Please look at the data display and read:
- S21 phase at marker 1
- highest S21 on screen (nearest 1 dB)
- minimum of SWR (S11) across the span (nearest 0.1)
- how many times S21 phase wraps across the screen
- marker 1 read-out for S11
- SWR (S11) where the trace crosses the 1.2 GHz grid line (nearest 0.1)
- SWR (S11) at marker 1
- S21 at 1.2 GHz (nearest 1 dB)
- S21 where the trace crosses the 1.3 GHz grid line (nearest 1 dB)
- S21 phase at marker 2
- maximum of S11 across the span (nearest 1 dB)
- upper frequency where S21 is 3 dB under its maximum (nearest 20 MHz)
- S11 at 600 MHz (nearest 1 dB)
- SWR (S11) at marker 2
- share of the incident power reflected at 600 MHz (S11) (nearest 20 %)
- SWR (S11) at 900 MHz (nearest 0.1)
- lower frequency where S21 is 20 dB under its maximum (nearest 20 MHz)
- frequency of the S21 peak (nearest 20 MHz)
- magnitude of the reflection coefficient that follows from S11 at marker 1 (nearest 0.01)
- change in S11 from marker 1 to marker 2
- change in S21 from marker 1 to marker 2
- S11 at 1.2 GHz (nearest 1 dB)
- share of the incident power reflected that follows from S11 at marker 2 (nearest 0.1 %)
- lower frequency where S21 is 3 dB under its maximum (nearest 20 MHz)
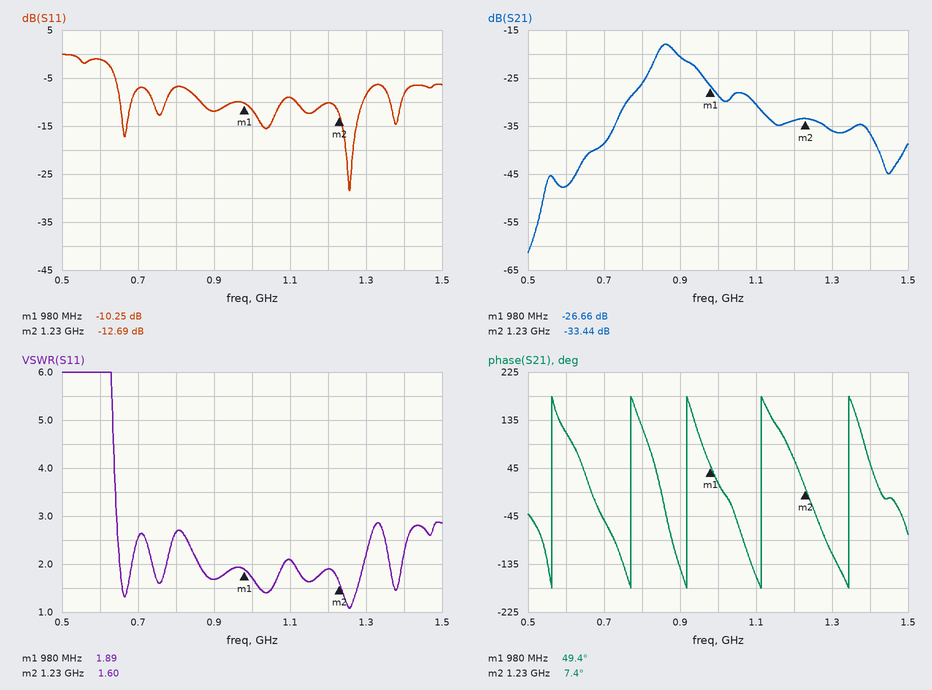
49.4°
-18 dB
1.1
5
-10.25 dB
1.9
1.89
-34 dB
-36 dB
7.4°
0 dB
900 MHz
-1 dB
1.60
80 %
1.7
700 MHz
860 MHz
0.31
-2.44 dB
-6.78 dB
-10 dB
5.4 %
840 MHz
